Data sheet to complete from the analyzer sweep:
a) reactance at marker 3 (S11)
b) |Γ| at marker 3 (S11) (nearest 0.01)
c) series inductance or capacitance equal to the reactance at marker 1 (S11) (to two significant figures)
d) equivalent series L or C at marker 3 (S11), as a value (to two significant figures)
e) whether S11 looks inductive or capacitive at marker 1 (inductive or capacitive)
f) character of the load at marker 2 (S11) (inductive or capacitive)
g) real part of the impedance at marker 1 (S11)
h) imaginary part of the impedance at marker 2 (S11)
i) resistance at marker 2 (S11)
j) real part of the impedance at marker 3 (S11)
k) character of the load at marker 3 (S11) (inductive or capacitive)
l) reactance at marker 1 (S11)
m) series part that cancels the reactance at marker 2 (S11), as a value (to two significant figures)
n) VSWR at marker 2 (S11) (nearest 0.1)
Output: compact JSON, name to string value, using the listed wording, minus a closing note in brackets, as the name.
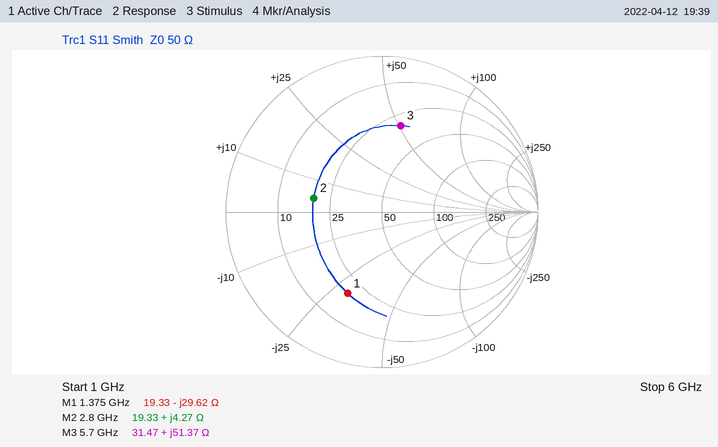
{"reactance at marker 3": "+51.37 Ω", "|Γ| at marker 3 (S11)": "0.57", "series inductance or capacitance equal to the reactance at marker 1 (S11)": "3.9 pF", "equivalent series L or C at marker 3 (S11), as a value": "1.4 nH", "whether S11 looks inductive or capacitive at marker 1": "capacitive", "character of the load at marker 2 (S11)": "inductive", "real part of the impedance at marker 1": "19.33 Ω", "imaginary part of the impedance at marker 2": "+4.27 Ω", "resistance at marker 2": "19.33 Ω", "real part of the impedance at marker 3": "31.47 Ω", "character of the load at marker 3 (S11)": "inductive", "reactance at marker 1": "-29.62 Ω", "series part that cancels the reactance at marker 2 (S11), as a value": "13 pF", "VSWR at marker 2 (S11)": "2.6"}
